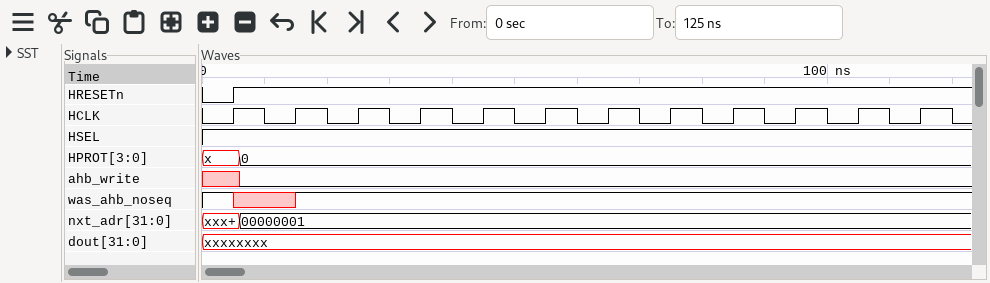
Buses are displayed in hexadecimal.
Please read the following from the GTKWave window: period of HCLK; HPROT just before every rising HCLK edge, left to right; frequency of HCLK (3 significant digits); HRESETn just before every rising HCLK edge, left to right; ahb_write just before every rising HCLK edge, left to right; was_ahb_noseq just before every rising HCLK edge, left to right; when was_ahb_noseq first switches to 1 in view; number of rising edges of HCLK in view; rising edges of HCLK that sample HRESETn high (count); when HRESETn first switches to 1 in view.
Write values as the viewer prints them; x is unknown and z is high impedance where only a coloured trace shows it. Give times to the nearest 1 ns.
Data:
10 ns
x, 0, 0, 0, 0, 0, 0, 0, 0, 0, 0, 0
100 MHz
0 1 1 1 1 1 1 1 1 1 1 1
x 0 0 0 0 0 0 0 0 0 0 0
1 x 1 1 1 1 1 1 1 1 1 1
15 ns
12
11
5 ns
